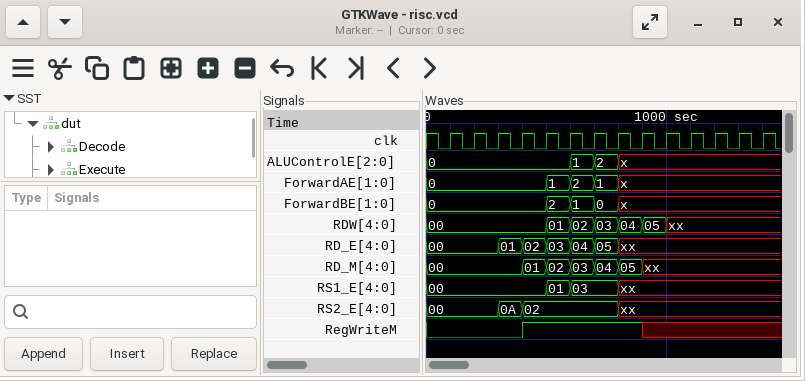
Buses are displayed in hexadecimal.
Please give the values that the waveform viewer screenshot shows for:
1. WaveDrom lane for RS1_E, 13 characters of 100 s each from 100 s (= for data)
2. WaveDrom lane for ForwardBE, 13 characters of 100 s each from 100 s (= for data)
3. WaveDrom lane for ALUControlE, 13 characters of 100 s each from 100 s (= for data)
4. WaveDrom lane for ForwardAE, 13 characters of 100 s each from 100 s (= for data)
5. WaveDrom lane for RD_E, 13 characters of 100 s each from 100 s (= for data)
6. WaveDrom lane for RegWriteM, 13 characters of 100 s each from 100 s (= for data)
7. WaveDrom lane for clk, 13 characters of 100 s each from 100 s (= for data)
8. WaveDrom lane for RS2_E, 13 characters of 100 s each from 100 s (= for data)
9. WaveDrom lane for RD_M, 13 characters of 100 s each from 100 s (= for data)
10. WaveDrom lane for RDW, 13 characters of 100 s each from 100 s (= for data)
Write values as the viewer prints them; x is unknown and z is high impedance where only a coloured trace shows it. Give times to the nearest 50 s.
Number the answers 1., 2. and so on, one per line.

1. {name: 'RS1_E', wave: '=...==.x.....', data: '00 01 03'}
2. {name: 'ForwardBE', wave: '=...===x.....', data: '0 2 1 0'}
3. {name: 'ALUControlE', wave: '=....==x.....', data: '0 1 2'}
4. {name: 'ForwardAE', wave: '=...===x.....', data: '0 1 2 1'}
5. {name: 'RD_E', wave: '=.=====x.....', data: '00 01 02 03 04 05'}
6. {name: 'RegWriteM', wave: '0..1....x....'}
7. {name: 'clk', wave: 'p............'}
8. {name: 'RS2_E', wave: '=.==...x.....', data: '00 0A 02'}
9. {name: 'RD_M', wave: '=..=====x....', data: '00 01 02 03 04 05'}
10. {name: 'RDW', wave: '=...=====x...', data: '00 01 02 03 04 05'}
